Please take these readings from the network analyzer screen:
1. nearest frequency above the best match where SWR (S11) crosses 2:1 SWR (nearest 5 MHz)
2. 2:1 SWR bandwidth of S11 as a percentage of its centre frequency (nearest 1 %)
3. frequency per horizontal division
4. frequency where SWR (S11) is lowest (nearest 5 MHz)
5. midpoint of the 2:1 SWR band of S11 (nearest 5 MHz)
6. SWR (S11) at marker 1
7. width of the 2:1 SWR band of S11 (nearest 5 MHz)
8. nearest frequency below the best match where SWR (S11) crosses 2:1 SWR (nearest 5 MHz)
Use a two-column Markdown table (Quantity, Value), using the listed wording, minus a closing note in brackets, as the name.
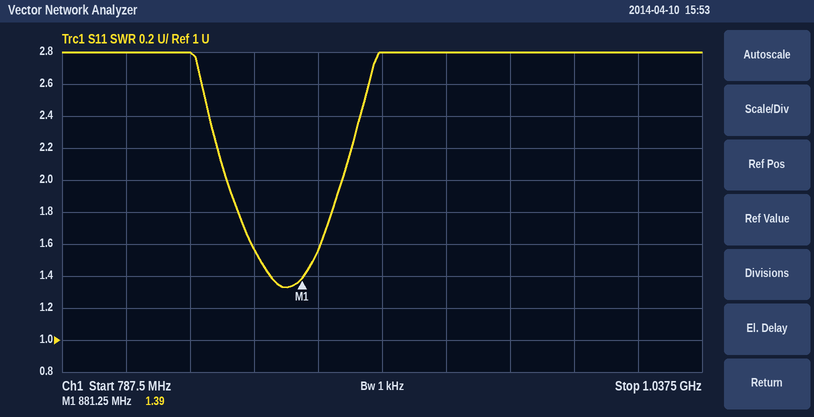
| Quantity | Value |
|---|---|
| nearest frequency above the best match where SWR (S11) crosses 2:1 SWR | 895 MHz |
| 2:1 SWR bandwidth of S11 as a percentage of its centre frequency | 5 % |
| frequency per horizontal division | 25 MHz |
| frequency where SWR (S11) is lowest | 875 MHz |
| midpoint of the 2:1 SWR band of S11 | 875 MHz |
| SWR (S11) at marker 1 | 1.39 |
| width of the 2:1 SWR band of S11 | 45 MHz |
| nearest frequency below the best match where SWR (S11) crosses 2:1 SWR | 850 MHz |
